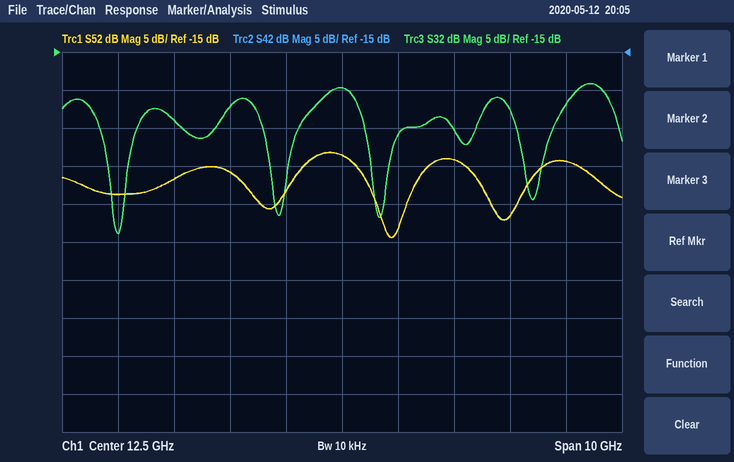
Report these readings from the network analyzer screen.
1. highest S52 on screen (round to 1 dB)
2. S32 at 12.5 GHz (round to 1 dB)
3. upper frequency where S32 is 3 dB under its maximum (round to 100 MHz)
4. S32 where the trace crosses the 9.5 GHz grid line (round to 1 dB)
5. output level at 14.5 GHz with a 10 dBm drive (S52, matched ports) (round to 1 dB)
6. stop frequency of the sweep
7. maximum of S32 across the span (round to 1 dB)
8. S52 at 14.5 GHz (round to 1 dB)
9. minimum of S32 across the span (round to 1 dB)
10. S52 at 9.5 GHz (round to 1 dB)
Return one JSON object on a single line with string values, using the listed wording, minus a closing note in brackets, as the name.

{"highest S52 on screen": "-28 dB", "S32 at 12.5 GHz": "-20 dB", "upper frequency where S32 is 3 dB under its maximum": "17.3 GHz", "S32 where the trace crosses the 9.5 GHz grid line": "-24 dB", "output level at 14.5 GHz with a 10 dBm drive (S52, matched ports)": "-19 dBm", "stop frequency of the sweep": "17.5 GHz", "maximum of S32 across the span": "-19 dB", "S52 at 14.5 GHz": "-29 dB", "minimum of S32 across the span": "-39 dB", "S52 at 9.5 GHz": "-32 dB"}
